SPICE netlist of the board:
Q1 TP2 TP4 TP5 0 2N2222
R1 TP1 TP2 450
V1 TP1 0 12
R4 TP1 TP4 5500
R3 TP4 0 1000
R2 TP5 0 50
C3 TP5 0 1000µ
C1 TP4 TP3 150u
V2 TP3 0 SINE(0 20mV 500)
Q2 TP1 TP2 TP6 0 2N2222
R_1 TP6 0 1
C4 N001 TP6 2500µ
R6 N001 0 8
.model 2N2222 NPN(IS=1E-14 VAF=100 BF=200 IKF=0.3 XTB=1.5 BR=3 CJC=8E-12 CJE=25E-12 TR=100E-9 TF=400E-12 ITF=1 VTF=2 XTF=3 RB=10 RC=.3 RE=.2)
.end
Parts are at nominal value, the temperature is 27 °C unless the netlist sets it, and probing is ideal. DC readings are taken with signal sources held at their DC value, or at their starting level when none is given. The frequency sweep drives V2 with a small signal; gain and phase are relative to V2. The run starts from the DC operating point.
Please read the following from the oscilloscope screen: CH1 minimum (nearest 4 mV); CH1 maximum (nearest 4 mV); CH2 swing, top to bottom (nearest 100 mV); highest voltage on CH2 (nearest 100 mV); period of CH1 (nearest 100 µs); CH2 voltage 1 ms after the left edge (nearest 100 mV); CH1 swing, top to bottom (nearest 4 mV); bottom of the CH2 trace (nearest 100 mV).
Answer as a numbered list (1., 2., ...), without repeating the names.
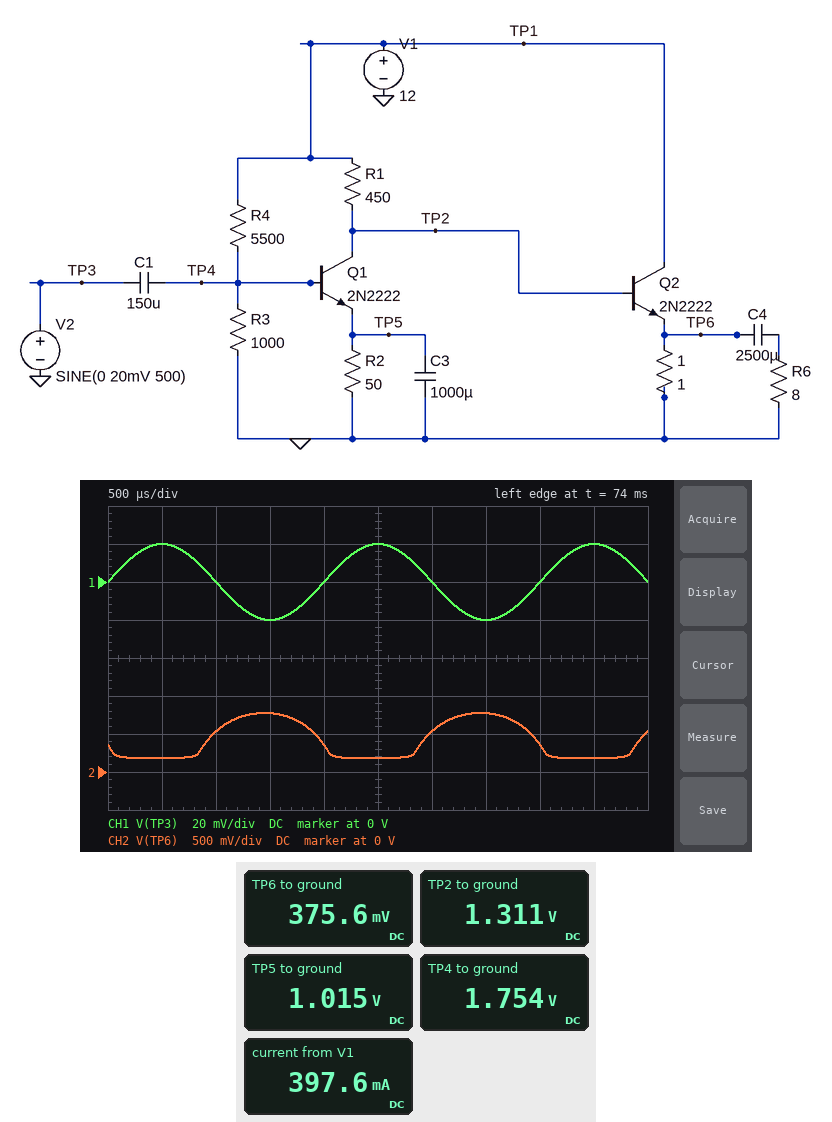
1. -20 mV
2. 20 mV
3. 600 mV
4. 800 mV
5. 2.0 ms
6. 500 mV
7. 40 mV
8. 200 mV
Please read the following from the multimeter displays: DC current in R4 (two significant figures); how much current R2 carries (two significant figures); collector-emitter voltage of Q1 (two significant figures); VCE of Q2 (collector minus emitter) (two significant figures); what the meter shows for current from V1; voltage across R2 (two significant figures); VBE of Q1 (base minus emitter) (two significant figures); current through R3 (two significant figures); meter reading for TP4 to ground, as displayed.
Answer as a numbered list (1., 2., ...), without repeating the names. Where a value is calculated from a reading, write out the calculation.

1. (12 V - 1.754 V) / 5.5 kΩ = 1.9 mA
2. (1.015 V) / 50 Ω = 20 mA
3. 1.311 V - 1.015 V = 300 mV
4. 12 V - 375.6 mV = 12 V
5. 397.6 mA
6. 1.015 V = 1.0 V
7. 1.754 V - 1.015 V = 740 mV
8. (1.754 V) / 1 kΩ = 1.8 mA
9. 1.754 V
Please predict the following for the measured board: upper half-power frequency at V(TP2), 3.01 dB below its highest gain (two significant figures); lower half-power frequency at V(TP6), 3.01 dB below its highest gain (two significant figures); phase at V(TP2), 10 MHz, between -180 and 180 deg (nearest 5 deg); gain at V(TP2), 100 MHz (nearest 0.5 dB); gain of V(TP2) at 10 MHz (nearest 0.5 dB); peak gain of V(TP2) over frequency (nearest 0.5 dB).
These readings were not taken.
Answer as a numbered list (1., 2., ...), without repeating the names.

1. 5.2 MHz
2. 100 Hz
3. 120 deg
4. 8.5 dB
5. 26.5 dB
6. 33.5 dB
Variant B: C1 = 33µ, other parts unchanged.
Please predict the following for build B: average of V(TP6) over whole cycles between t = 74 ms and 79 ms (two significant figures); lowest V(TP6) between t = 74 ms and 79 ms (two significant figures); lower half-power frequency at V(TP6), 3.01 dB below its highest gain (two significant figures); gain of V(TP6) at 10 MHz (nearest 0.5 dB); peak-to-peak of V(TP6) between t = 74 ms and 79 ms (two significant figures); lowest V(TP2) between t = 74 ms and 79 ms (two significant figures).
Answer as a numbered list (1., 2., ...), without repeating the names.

1. 460 mV
2. 170 mV
3. 120 Hz
4. 23.0 dB
5. 620 mV
6. 990 mV
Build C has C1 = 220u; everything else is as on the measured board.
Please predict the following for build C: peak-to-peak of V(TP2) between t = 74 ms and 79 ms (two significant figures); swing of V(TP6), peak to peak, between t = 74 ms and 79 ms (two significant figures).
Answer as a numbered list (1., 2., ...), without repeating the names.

1. 890 mV
2. 580 mV
